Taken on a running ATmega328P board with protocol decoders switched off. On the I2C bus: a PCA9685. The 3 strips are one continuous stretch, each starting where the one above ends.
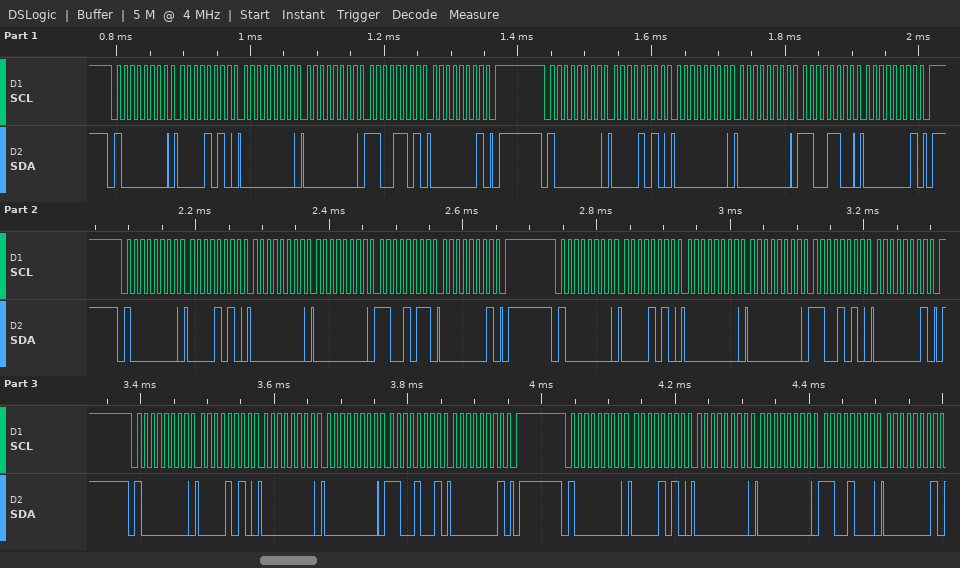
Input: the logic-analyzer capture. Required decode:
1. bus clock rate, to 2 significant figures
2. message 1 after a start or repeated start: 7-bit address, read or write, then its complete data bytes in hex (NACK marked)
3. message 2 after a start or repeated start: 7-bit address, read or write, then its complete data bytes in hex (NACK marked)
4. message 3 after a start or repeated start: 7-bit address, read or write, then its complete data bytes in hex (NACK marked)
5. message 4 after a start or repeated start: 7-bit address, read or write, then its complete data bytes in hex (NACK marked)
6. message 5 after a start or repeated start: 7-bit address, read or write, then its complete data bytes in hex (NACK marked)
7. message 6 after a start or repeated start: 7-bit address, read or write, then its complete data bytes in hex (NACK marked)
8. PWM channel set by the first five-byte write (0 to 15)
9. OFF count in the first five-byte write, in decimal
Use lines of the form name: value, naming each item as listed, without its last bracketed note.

bus clock rate, to 2 significant figures: 100 kHz
message 1 after a start or repeated start: 7-bit address, read or write, then its complete data bytes in hex: 0x40 write: 0A 00 00 CD 01
message 2 after a start or repeated start: 7-bit address, read or write, then its complete data bytes in hex: 0x40 write: 0A 00 00 CC 01
message 3 after a start or repeated start: 7-bit address, read or write, then its complete data bytes in hex: 0x40 write: 0A 00 00 CB 01
message 4 after a start or repeated start: 7-bit address, read or write, then its complete data bytes in hex: 0x40 write: 0A 00 00 CA 01
message 5 after a start or repeated start: 7-bit address, read or write, then its complete data bytes in hex: 0x40 write: 0A 00 00 C9 01
message 6 after a start or repeated start: 7-bit address, read or write, then its complete data bytes in hex: 0x40 write: 0A 00 00 C8 01
PWM channel set by the first five-byte write: 1
OFF count in the first five-byte write, in decimal: 461
